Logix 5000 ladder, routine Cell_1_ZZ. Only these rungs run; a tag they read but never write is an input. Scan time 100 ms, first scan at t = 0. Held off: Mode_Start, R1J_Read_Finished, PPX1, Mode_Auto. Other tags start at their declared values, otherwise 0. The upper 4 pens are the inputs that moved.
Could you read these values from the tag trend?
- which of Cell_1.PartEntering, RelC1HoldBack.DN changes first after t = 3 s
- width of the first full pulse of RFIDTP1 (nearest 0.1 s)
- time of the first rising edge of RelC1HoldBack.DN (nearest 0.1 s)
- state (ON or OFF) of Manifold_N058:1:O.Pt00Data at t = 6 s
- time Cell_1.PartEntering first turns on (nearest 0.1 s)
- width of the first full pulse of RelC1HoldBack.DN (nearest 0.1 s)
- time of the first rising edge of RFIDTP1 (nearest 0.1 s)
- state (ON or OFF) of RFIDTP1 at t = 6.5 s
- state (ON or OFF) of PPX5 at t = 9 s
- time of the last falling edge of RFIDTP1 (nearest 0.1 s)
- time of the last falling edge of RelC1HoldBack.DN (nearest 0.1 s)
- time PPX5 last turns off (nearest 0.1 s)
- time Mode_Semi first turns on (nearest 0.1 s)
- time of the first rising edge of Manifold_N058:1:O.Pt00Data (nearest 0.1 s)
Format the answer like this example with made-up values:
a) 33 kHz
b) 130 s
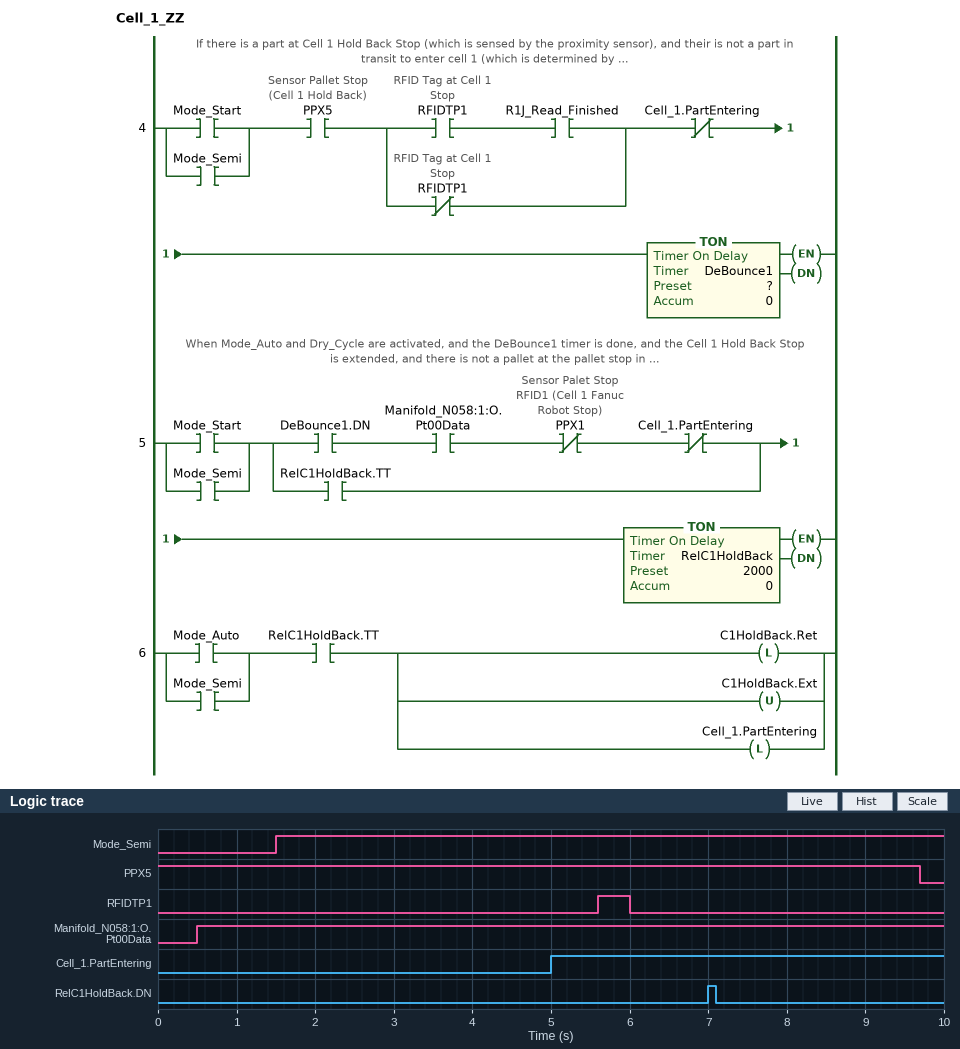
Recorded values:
a) Cell_1.PartEntering
b) 0.4 s
c) 7.0 s
d) ON
e) 5.0 s
f) 0.1 s
g) 5.6 s
h) OFF
i) ON
j) 6.0 s
k) 7.1 s
l) 9.7 s
m) 1.5 s
n) 0.5 s
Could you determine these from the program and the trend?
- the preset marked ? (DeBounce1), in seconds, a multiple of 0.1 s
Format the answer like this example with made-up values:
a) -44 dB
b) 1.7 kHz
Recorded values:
a) 3.5 s
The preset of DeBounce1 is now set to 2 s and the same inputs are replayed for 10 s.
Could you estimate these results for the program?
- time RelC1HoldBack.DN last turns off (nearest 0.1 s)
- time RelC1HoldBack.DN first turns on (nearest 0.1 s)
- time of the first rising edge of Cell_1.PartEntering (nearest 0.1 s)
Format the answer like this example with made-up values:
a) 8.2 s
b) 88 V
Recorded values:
a) 5.6 s
b) 5.5 s
c) 3.5 s
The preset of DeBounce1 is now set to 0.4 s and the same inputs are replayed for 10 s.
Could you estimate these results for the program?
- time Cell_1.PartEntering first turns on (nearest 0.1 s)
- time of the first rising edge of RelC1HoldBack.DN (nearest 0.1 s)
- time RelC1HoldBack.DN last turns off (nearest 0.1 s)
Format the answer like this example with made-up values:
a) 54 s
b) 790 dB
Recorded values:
a) 1.9 s
b) 3.9 s
c) 4.0 s
